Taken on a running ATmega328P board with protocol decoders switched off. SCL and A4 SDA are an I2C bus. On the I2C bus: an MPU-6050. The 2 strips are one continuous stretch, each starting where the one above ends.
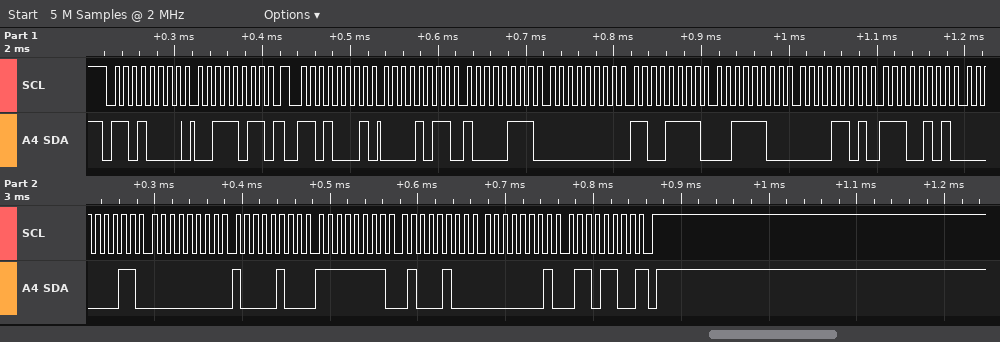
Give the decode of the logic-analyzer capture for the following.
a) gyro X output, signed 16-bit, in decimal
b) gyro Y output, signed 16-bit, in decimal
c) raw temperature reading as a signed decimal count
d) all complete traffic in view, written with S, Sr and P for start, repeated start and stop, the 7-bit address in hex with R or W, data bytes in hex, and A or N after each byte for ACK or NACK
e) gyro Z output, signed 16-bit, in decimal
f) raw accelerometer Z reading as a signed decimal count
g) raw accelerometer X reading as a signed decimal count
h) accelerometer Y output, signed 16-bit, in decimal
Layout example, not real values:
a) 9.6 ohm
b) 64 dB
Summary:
a) 132
b) -188
c) -6909
d) S 68W A 3B A Sr 68R A 0B A 87 A 00 A CF A 3C A 0D A E5 A 03 A 00 A 84 A FF A 44 A 01 A 6C N P
e) 364
f) 15373
g) 2951
h) 207
